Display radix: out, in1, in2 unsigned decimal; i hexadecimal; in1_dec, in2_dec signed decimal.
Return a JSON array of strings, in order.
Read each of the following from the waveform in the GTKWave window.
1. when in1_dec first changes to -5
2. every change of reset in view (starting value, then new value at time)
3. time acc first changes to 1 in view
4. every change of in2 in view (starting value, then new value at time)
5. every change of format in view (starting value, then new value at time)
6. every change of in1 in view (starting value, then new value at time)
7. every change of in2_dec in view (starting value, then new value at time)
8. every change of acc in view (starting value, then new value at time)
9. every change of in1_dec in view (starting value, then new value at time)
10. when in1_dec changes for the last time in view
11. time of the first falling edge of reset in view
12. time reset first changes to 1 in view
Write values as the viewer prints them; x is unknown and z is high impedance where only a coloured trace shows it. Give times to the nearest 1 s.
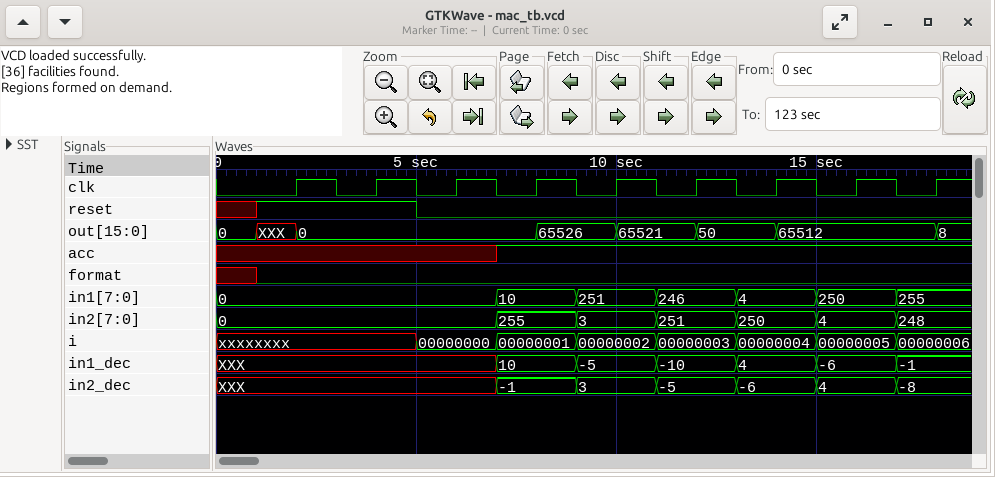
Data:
["9 s", "x, 1 at 1 s, 0 at 5 s", "7 s", "0, 255 at 7 s, 3 at 9 s, 251 at 11 s, 250 at 13 s, 4 at 15 s, 248 at 17 s", "x, 0 at 1 s", "0, 10 at 7 s, 251 at 9 s, 246 at 11 s, 4 at 13 s, 250 at 15 s, 255 at 17 s", "XXX, -1 at 7 s, 3 at 9 s, -5 at 11 s, -6 at 13 s, 4 at 15 s, -8 at 17 s", "x, 1 at 7 s", "XXX, 10 at 7 s, -5 at 9 s, -10 at 11 s, 4 at 13 s, -6 at 15 s, -1 at 17 s", "17 s", "5 s", "1 s"]
